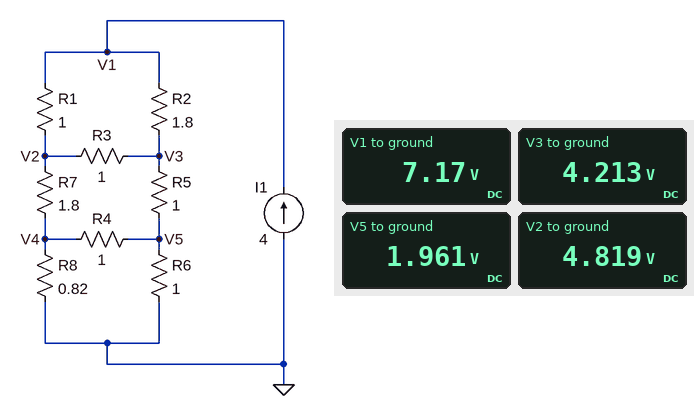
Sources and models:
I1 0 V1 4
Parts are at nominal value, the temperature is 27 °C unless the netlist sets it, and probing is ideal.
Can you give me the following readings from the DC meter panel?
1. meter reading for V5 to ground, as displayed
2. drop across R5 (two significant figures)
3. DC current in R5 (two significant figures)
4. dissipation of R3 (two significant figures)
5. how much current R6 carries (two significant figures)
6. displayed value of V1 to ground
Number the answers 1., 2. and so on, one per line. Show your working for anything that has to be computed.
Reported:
1. 1.961 V
2. 4.213 V - 1.961 V = 2.3 V
3. (4.213 V - 1.961 V) / 1 Ω = 2.3 A
4. (4.819 V - 4.213 V)^2 / 1 Ω = 370 mW
5. (1.961 V) / 1 Ω = 2.0 A
6. 7.17 V
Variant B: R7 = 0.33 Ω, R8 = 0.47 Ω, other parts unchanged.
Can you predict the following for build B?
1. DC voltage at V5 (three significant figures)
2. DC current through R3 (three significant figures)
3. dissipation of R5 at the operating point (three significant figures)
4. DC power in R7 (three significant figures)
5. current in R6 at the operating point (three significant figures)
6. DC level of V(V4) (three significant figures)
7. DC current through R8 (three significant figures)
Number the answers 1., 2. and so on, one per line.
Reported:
1. 1.24 V
2. 185 mA
3. 1.39 W
4. 2.63 W
5. 1.24 A
6. 1.30 V
7. 2.76 A
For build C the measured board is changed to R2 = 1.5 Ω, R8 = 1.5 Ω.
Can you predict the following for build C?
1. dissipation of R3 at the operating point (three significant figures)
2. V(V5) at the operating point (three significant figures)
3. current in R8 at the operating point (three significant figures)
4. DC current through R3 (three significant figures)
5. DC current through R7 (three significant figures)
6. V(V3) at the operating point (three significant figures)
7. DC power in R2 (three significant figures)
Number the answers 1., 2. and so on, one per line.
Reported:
1. 309 mW
2. 2.39 V
3. 1.61 A
4. 556 mA
5. 1.62 A
6. 4.77 V
7. 4.98 W
